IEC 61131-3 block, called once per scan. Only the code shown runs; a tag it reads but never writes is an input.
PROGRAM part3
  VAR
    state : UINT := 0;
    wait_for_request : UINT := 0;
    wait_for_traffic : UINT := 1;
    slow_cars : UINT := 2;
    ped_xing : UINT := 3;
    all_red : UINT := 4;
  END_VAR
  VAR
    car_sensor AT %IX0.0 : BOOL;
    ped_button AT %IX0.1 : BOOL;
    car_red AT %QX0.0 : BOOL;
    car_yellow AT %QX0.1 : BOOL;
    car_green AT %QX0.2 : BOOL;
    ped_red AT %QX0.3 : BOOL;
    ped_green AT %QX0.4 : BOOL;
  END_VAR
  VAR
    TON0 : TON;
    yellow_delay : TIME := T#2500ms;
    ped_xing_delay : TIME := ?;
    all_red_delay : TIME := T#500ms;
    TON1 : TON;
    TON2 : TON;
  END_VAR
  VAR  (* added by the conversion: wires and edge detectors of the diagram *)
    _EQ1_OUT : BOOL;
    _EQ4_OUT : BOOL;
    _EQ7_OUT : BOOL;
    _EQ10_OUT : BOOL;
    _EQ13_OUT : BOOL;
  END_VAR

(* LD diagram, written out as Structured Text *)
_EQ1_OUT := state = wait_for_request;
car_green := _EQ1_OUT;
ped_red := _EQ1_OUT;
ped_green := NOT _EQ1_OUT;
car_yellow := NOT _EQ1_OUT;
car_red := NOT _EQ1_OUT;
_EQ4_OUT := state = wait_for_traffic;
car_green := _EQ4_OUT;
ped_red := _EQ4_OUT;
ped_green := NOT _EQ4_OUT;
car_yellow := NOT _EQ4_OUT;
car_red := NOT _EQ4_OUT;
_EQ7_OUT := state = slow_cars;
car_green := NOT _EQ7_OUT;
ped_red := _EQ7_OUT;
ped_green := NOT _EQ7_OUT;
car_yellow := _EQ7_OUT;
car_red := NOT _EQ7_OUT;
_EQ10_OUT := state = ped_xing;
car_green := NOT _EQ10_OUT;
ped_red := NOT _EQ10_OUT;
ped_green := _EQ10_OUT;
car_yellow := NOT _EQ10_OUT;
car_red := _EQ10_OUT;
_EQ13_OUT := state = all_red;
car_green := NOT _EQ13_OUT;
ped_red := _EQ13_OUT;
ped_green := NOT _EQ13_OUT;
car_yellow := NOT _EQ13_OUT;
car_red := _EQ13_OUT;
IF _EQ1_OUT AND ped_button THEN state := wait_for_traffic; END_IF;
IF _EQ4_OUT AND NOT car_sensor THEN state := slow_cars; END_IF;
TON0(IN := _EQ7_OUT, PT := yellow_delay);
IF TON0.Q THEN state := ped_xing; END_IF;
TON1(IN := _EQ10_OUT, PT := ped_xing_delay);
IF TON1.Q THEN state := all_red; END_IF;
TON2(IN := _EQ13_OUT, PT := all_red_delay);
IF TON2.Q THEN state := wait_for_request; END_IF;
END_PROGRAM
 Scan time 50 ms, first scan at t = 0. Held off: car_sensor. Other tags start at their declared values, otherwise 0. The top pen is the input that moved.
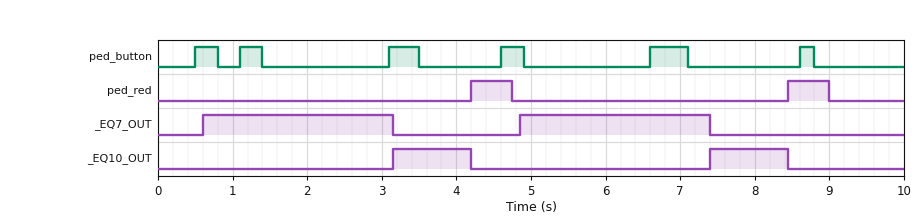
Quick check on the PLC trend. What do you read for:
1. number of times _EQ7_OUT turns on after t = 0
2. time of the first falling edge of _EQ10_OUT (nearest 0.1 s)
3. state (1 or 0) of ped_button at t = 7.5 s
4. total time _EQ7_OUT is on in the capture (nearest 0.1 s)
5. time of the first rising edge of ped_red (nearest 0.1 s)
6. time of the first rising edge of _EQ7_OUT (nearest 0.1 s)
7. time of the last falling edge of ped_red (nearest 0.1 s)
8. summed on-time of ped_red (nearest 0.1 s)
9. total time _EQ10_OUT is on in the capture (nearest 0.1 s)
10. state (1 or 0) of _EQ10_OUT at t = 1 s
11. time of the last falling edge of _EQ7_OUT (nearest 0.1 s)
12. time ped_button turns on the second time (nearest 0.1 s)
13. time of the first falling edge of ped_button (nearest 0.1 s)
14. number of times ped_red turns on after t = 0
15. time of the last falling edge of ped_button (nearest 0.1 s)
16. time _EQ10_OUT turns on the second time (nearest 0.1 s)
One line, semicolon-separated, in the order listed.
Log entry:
2; 4.2 s; 0; 5.1 s; 4.2 s; 0.6 s; 9.0 s; 1.1 s; 2.1 s; 0; 7.4 s; 1.1 s; 0.8 s; 2; 8.8 s; 7.4 s
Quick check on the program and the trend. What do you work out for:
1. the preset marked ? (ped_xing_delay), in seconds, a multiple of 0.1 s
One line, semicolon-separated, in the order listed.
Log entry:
1.0 s
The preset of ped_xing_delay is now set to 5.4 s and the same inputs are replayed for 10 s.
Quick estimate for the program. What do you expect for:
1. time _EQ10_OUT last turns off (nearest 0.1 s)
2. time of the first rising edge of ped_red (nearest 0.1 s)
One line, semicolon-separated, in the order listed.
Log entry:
8.6 s; 8.6 s
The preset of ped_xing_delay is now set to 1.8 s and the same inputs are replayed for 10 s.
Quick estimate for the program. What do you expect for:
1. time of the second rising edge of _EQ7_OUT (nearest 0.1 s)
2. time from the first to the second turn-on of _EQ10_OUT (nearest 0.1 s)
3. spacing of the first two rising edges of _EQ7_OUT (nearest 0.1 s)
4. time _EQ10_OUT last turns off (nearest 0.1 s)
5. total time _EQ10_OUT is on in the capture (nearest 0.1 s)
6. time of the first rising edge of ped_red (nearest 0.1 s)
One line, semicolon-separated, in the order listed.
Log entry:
6.7 s; 6.1 s; 6.1 s; 5.0 s; 2.6 s; 5.0 s
